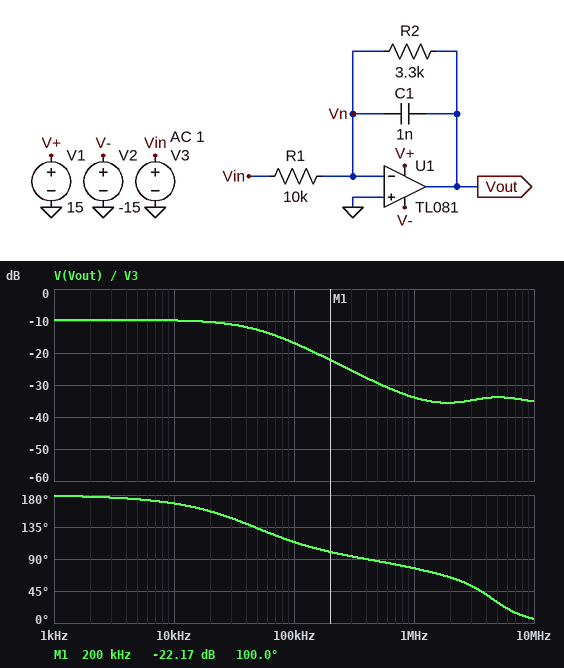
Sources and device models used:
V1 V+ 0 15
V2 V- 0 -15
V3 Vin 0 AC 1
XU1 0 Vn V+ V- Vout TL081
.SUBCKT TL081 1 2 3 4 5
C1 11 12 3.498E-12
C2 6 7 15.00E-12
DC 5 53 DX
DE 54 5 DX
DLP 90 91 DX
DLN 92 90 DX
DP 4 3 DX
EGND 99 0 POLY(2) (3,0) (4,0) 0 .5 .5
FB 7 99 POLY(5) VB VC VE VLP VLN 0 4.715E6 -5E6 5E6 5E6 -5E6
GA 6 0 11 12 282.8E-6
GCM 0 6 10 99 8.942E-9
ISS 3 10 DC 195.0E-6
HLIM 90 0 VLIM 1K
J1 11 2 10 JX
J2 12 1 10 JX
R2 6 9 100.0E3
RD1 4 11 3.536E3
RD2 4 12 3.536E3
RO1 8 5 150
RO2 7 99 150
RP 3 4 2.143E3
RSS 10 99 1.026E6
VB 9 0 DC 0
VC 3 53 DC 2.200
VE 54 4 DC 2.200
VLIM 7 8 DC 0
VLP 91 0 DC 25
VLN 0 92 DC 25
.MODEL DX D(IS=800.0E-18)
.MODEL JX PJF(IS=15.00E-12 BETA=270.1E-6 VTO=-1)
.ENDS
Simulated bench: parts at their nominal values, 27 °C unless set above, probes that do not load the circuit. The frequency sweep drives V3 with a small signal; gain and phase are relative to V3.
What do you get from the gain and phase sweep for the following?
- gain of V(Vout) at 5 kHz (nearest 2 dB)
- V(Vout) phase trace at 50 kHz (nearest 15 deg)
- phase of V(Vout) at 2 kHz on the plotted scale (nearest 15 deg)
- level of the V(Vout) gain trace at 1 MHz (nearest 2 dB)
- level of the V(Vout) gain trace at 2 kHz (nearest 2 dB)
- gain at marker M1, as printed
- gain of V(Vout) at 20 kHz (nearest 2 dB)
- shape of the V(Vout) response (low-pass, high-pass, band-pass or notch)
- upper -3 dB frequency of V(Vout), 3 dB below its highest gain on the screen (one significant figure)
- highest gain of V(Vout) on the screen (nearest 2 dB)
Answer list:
-10 dB
135 deg
180 deg
-34 dB
-10 dB
-22.17 dB
-10 dB
low-pass
50 kHz
-10 dB
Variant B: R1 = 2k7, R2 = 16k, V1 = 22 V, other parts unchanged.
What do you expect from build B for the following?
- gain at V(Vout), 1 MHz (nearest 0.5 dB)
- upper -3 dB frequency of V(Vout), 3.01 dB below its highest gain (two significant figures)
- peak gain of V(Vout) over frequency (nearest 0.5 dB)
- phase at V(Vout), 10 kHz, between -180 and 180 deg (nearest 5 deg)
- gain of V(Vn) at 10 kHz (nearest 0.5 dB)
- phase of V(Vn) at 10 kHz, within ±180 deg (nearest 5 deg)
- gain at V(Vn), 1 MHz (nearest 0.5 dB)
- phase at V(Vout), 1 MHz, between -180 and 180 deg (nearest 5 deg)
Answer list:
-22.5 dB
9.8 kHz
15.5 dB
135 deg
-38.5 dB
45 deg
-32.5 dB
75 deg
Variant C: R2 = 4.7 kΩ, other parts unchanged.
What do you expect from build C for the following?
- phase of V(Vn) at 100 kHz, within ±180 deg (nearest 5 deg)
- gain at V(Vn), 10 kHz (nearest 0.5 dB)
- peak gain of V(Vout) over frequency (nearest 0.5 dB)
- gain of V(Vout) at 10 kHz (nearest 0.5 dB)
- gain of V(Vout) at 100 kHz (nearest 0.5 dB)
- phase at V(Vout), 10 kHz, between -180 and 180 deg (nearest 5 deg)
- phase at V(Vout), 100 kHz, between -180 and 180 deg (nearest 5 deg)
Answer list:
25 deg
-57.5 dB
-6.5 dB
-7.0 dB
-16.5 dB
165 deg
105 deg
